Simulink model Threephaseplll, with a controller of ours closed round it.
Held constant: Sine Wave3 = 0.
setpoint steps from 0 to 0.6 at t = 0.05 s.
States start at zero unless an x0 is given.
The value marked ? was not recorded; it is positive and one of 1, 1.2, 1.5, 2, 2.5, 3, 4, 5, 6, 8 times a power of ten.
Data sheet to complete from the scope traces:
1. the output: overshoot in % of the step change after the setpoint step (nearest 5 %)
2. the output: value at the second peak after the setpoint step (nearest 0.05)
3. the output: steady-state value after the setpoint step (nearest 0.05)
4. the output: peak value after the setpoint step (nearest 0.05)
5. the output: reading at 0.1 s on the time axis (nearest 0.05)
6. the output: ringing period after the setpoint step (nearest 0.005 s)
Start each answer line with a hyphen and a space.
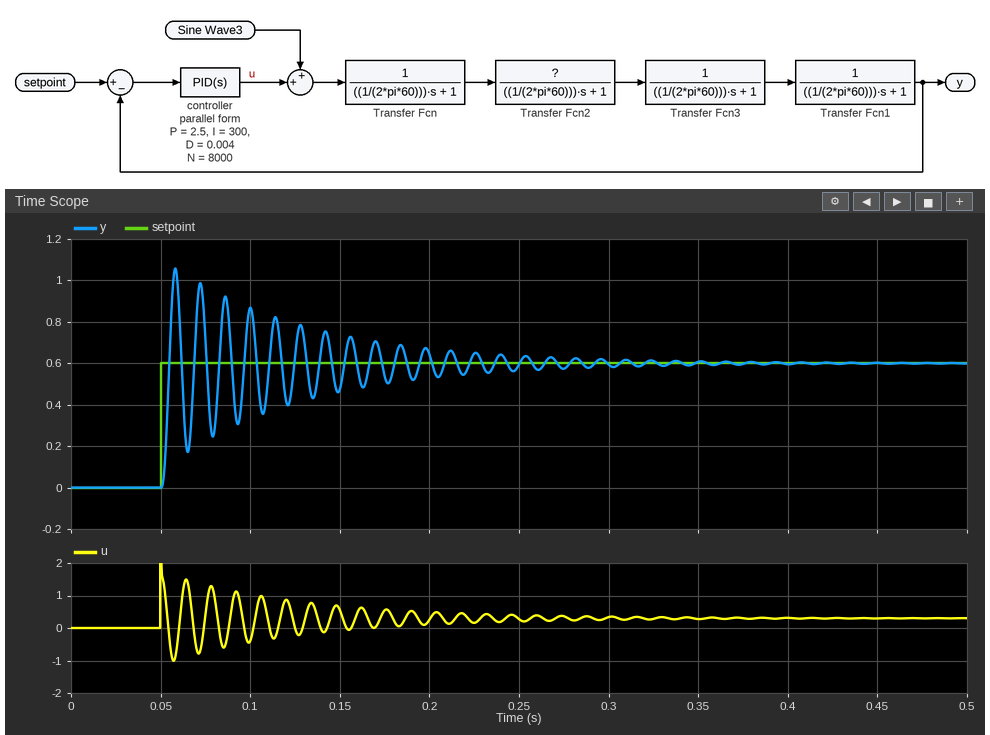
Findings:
- 75 %
- 1.00
- 0.60
- 1.05
- 0.85
- 0.015 s
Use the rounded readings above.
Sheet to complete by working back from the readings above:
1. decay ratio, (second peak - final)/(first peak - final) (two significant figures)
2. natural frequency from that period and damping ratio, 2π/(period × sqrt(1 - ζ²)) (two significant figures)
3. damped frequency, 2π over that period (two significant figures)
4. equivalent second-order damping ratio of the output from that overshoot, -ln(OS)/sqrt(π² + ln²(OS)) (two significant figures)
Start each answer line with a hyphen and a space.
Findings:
- 0.89
- 420 rad/s
- 420 rad/s
- 0.091
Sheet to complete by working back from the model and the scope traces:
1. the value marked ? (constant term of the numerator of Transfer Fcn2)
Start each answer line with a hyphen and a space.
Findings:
- 2
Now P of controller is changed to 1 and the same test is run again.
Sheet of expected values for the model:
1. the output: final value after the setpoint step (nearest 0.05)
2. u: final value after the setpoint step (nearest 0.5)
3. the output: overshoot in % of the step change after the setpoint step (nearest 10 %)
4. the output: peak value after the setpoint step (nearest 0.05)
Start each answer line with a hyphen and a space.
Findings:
- 0.60
- 0.5
- 40 %
- 0.85
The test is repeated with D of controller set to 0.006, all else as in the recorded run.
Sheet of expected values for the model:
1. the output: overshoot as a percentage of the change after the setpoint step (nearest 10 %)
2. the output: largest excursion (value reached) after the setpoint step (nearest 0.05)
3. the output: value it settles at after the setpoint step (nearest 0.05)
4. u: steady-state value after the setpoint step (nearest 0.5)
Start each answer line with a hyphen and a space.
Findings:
- 60 %
- 1.00
- 0.60
- 0.5
